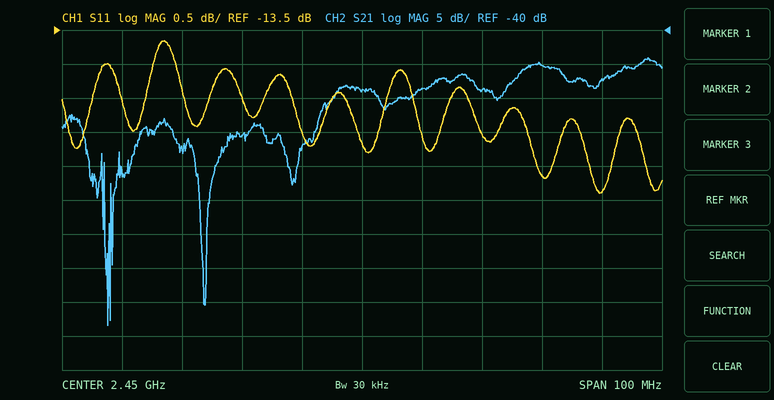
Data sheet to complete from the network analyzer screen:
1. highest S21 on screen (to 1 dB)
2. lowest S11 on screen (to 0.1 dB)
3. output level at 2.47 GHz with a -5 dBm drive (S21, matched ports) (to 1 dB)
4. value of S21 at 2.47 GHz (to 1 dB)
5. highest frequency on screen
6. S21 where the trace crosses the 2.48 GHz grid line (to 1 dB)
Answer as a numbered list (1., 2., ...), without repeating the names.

1. -44 dB
2. -15.9 dB
3. -54 dBm
4. -49 dB
5. 2.5 GHz
6. -45 dB
